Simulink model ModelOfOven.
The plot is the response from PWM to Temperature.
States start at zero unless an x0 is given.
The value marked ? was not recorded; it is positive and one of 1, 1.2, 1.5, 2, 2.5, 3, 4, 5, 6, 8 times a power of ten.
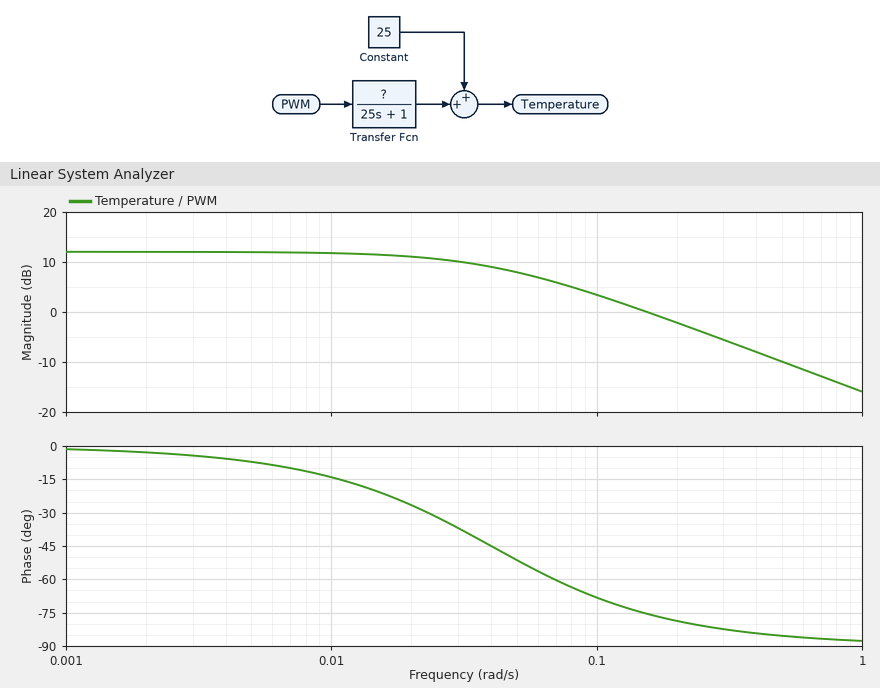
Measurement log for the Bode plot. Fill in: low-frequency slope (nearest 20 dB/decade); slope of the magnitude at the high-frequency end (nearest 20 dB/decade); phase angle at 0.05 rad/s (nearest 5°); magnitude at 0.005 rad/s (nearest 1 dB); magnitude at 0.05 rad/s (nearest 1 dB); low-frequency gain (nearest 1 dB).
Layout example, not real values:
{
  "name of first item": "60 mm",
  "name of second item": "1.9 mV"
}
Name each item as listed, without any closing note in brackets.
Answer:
{
  "low-frequency slope": "0 dB/decade",
  "slope of the magnitude at the high-frequency end": "-20 dB/decade",
  "phase angle at 0.05 rad/s": "-50°",
  "magnitude at 0.005 rad/s": "12 dB",
  "magnitude at 0.05 rad/s": "8 dB",
  "low-frequency gain": "12 dB"
}
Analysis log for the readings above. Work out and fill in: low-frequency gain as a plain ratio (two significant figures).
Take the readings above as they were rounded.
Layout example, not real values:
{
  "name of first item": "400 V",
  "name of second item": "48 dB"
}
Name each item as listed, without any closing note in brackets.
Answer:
{
  "low-frequency gain as a plain ratio": "4.0"
}
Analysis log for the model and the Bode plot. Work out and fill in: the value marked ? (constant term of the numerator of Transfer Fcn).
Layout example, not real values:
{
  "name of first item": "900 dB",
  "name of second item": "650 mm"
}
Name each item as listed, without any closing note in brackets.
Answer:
{
  "the value marked ?": "4"
}
